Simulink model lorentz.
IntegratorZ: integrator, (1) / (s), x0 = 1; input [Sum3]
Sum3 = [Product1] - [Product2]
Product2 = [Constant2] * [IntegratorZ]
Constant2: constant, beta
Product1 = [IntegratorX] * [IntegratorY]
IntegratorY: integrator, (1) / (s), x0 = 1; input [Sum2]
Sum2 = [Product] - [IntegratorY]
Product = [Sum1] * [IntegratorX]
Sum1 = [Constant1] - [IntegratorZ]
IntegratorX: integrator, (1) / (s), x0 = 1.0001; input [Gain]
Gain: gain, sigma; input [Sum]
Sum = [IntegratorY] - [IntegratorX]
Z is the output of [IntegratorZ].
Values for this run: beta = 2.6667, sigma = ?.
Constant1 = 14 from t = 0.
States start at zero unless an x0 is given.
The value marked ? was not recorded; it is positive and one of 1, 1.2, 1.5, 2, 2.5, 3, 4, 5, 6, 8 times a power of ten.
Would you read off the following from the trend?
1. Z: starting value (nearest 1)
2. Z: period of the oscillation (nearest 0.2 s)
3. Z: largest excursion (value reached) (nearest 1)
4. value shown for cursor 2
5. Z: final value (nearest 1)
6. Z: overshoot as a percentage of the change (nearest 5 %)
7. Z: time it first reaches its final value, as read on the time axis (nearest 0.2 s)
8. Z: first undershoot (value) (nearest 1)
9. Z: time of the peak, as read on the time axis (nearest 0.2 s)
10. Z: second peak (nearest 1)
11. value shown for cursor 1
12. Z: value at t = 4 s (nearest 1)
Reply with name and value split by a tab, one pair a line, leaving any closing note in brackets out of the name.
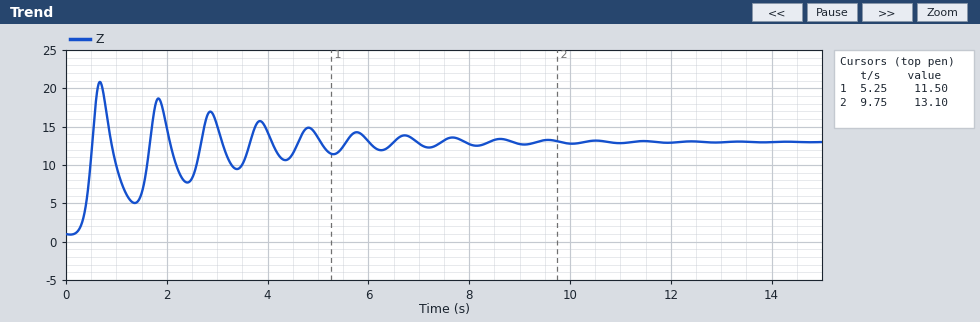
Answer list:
Z: starting value	1
Z: period of the oscillation	1.2 s
Z: largest excursion (value reached)	21
value shown for cursor 2	13.10
Z: final value	13
Z: overshoot as a percentage of the change	65 %
Z: time it first reaches its final value, as read on the time axis	0.6 s
Z: first undershoot (value)	5
Z: time of the peak, as read on the time axis	0.6 s
Z: second peak	19
value shown for cursor 1	11.50
Z: value at t = 4 s	14
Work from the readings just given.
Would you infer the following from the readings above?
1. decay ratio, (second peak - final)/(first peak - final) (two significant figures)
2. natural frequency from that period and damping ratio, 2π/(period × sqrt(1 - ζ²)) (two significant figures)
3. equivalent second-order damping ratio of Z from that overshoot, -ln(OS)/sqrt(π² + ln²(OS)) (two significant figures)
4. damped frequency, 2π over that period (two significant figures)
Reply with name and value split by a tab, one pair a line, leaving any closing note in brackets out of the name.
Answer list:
decay ratio, (second peak - final)/(first peak - final)	0.75
natural frequency from that period and damping ratio, 2π/(period × sqrt(1 - ζ²))	5.3 rad/s
equivalent second-order damping ratio of Z from that overshoot, -ln(OS)/sqrt(π² + ln²(OS))	0.14
damped frequency, 2π over that period	5.2 rad/s
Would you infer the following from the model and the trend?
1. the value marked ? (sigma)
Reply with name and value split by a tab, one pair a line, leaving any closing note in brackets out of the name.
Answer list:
the value marked ?	5
